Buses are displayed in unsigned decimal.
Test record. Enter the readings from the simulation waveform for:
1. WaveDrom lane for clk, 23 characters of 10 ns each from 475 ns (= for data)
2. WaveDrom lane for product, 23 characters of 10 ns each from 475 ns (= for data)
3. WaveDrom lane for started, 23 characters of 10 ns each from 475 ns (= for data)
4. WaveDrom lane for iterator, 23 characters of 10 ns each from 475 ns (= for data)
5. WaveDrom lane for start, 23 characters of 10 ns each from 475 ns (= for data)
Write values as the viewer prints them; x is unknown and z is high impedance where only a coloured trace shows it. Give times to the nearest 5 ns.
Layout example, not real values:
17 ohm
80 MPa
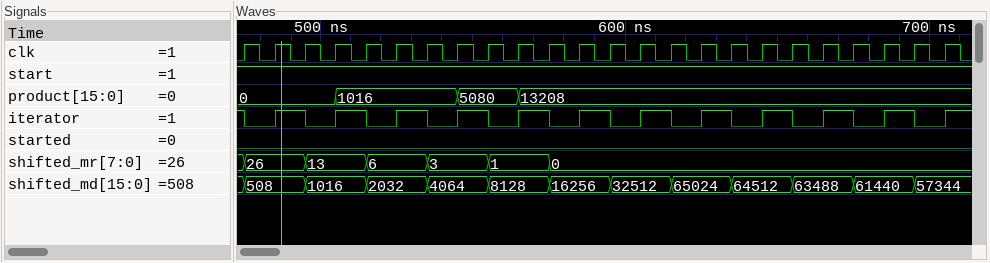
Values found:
{name: 'clk', wave: 'p......................'}
{name: 'product', wave: '=..=...=.=.............', data: '0 1016 5080 13208'}
{name: 'started', wave: '0......................'}
{name: 'iterator', wave: '01010101010101010101010'}
{name: 'start', wave: '1......................'}
